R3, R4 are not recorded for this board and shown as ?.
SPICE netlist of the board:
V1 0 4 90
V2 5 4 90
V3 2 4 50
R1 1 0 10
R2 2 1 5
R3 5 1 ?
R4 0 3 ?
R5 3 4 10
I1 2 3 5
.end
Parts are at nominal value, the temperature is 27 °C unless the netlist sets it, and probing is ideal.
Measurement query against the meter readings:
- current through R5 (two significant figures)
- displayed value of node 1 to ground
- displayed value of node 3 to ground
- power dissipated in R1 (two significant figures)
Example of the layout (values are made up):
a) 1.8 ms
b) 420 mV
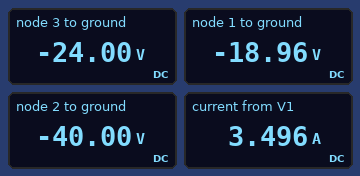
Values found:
a) 6.6 A
b) -18.96 V
c) -24.00 V
d) 36 W
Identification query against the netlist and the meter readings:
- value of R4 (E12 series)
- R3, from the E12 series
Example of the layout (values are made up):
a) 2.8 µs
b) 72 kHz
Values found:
a) 15 Ω
b) 8.2 Ω
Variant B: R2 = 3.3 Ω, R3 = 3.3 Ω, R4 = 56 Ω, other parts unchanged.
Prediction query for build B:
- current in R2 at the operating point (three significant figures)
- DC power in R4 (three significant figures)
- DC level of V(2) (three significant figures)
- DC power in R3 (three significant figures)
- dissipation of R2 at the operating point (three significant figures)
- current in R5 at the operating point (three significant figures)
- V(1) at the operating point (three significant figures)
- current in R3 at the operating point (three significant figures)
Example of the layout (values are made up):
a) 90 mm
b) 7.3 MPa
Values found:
a) 6.92 A
b) 20.6 W
c) -40.0 V
d) 89.3 W
e) 158 W
f) 5.61 A
g) -17.2 V
h) 5.20 A
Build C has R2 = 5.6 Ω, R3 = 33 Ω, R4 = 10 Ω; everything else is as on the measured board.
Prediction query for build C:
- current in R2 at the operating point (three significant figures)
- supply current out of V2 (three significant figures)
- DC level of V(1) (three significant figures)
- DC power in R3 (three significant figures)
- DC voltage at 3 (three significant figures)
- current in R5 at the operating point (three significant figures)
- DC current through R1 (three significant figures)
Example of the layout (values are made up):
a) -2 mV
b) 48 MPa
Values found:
a) 3.01 A
b) 701 mA
c) -23.1 V
d) 16.2 W
e) -20.0 V
f) 7.00 A
g) 2.31 A
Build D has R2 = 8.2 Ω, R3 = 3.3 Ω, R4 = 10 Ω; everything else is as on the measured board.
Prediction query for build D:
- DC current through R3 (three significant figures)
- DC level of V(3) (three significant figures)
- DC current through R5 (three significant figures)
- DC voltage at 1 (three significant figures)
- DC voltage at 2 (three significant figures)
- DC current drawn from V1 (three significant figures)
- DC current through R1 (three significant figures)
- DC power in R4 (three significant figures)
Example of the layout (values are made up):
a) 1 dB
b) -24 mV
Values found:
a) 2.82 A
b) -20.0 V
c) 7.00 A
d) -9.29 V
e) -40.0 V
f) 2.93 A
g) 929 mA
h) 40.0 W
